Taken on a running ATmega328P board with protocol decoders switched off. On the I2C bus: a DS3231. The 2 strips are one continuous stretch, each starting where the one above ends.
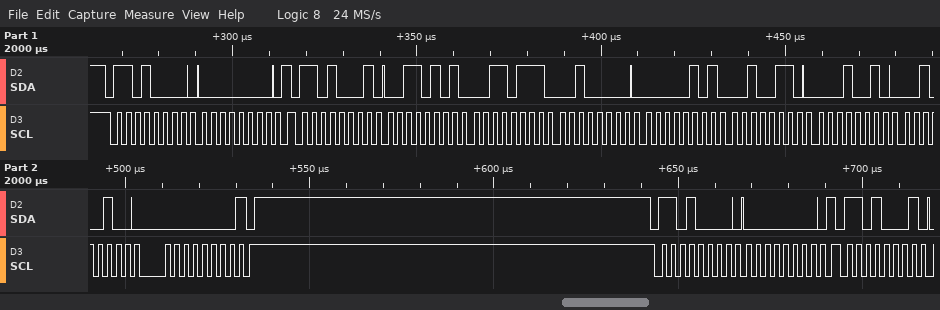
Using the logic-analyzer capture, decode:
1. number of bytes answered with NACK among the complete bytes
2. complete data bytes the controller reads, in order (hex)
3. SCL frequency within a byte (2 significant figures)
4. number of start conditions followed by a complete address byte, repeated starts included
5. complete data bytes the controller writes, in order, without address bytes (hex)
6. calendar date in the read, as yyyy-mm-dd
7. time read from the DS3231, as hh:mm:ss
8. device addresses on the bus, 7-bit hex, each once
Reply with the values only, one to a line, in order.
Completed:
1
35 37 20 05 26 12 24 00
400 kHz
4
00 00
2024-12-26
20:37:35
0x68
